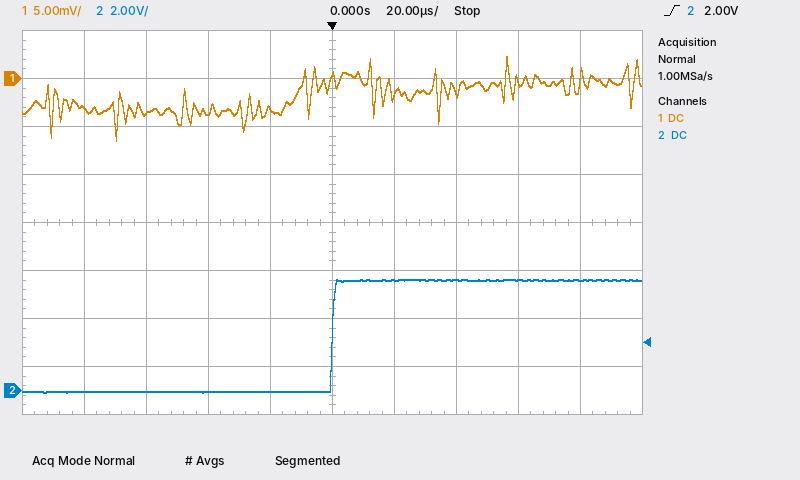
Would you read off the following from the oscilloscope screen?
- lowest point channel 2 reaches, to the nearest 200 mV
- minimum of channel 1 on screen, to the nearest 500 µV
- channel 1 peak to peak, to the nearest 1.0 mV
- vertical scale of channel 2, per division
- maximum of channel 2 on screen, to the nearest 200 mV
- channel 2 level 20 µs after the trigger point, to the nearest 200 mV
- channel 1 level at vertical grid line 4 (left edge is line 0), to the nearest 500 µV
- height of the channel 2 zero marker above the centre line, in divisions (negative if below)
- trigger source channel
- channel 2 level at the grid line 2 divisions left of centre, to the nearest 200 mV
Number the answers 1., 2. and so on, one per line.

1. 0.0 V
2. -6.5 mV
3. 9.0 mV
4. 2 V
5. 4.6 V
6. 4.6 V
7. -3.0 mV
8. -3.5 div
9. channel 2
10. 0.0 V
